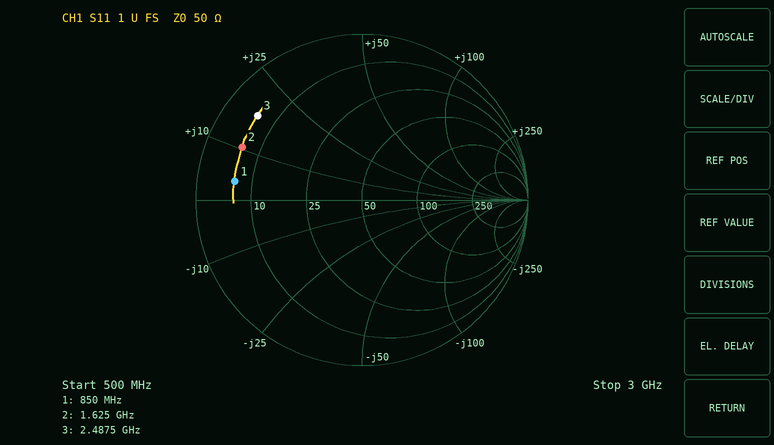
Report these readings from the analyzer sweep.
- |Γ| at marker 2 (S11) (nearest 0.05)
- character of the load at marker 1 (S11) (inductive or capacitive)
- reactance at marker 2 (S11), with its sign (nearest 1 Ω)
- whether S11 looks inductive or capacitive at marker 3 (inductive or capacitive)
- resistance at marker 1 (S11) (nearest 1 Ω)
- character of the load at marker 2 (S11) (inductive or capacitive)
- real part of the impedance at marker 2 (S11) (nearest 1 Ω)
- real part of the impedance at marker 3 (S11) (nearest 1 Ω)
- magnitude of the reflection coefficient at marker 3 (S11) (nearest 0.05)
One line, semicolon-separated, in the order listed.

0.80; inductive; +10 Ω; inductive; 6 Ω; inductive; 6 Ω; 6 Ω; 0.80
